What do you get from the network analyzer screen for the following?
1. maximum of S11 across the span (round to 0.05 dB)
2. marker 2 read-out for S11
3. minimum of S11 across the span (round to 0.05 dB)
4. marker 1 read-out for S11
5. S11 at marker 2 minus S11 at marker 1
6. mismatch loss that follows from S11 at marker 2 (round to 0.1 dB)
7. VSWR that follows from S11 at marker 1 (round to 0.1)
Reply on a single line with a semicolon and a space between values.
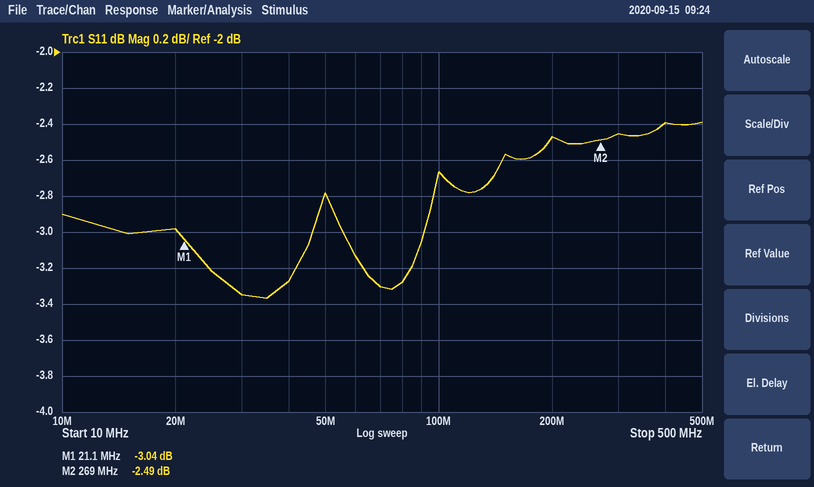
-2.40 dB; -2.49 dB; -3.35 dB; -3.04 dB; 0.55 dB; 3.6 dB; 5.8
